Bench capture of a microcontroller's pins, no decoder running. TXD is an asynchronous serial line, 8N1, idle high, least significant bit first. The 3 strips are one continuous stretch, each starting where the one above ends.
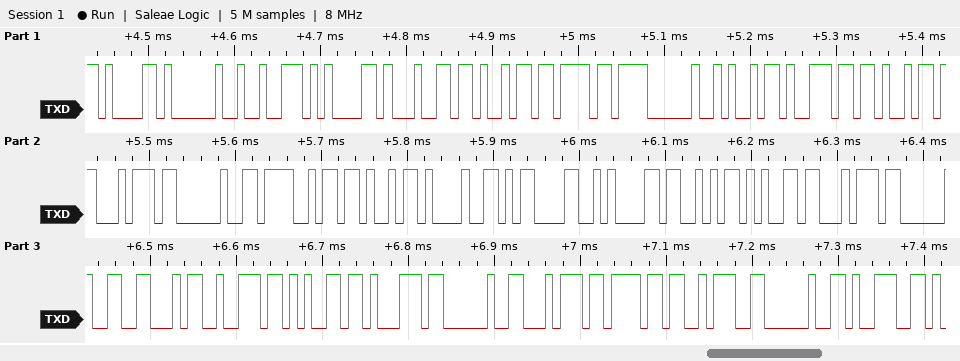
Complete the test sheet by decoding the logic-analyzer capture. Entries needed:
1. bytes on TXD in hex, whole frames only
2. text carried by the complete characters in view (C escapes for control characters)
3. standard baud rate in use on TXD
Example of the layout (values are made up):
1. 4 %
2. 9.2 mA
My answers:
1. 0x61 0x20 0x72 0x61 0x64 0x69 0x6F 0x20 0x69 0x6E 0x69 0x74 0x20 0x4F 0x4B 0x21 0x0D 0x0A 0x53 0x65 0x74 0x20 0x46 0x72 0x65 0x71 0x20 0x74 0x6F 0x3A 0x20 0x39
2. "a radio init OK!\r\nSet Freq to: 9"
3. 115200 baud
